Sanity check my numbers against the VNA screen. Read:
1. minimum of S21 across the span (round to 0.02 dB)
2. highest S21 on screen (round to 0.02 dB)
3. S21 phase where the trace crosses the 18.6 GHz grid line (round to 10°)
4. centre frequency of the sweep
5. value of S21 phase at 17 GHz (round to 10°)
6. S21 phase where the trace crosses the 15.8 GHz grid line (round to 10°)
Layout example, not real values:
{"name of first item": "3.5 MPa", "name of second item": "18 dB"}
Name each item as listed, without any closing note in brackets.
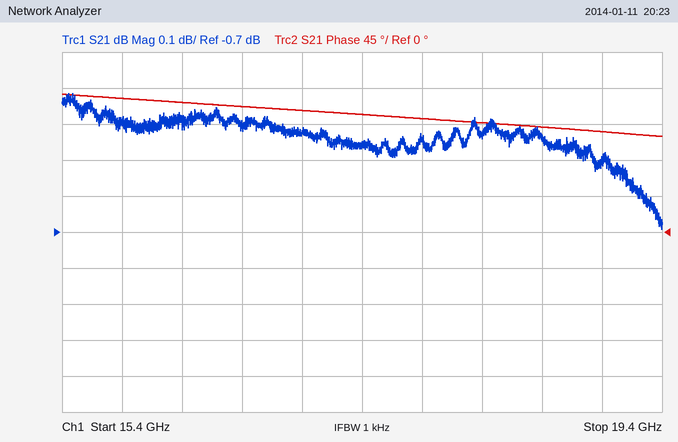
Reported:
{"minimum of S21 across the span": "-0.70 dB", "highest S21 on screen": "-0.32 dB", "S21 phase where the trace crosses the 18.6 GHz grid line": "130°", "centre frequency of the sweep": "17.4 GHz", "value of S21 phase at 17 GHz": "150°", "S21 phase where the trace crosses the 15.8 GHz grid line": "170°"}
